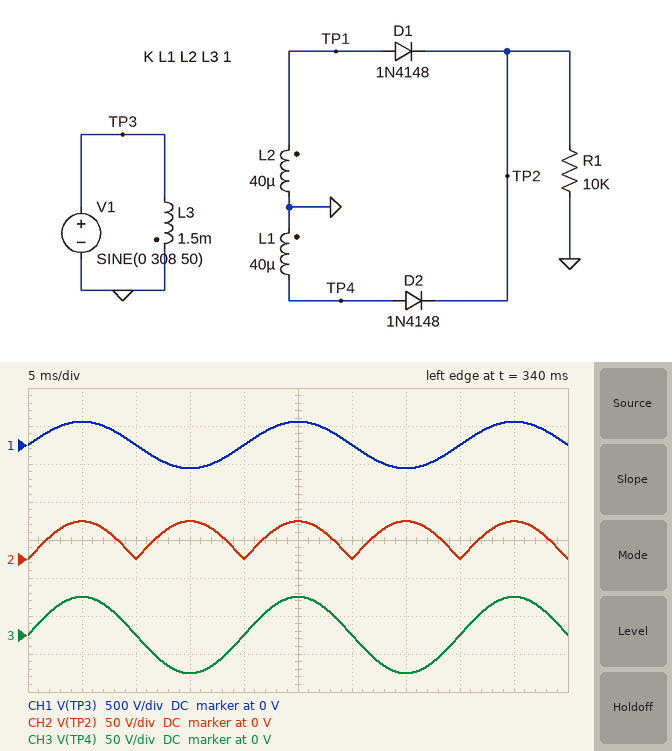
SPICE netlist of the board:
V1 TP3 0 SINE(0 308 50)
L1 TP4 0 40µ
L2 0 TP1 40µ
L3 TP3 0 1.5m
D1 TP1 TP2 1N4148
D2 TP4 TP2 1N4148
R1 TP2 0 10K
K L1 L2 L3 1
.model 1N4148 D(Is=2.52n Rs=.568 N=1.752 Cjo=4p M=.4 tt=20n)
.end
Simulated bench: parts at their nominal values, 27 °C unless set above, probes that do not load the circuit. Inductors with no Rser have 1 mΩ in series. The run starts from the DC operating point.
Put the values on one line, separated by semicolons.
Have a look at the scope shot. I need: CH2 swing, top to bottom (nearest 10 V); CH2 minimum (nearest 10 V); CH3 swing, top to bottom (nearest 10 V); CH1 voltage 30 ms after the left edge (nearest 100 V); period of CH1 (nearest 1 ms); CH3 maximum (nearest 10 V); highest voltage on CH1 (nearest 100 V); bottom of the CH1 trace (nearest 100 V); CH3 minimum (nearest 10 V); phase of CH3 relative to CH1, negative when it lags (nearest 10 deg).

50 V; 0 V; 100 V; 0 V; 20 ms; 50 V; 300 V; -300 V; -50 V; 0 deg
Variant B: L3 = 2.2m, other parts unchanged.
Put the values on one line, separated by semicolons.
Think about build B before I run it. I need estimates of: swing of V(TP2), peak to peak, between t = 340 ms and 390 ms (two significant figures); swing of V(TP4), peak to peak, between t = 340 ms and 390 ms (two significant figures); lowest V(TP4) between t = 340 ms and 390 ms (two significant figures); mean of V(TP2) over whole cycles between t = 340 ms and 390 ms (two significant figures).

41 V; 83 V; -42 V; 26 V
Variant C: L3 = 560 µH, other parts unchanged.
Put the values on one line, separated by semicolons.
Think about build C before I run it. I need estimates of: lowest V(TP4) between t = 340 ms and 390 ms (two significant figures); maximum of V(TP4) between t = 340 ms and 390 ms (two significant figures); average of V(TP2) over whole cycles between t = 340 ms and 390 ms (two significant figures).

-83 V; 82 V; 52 V
